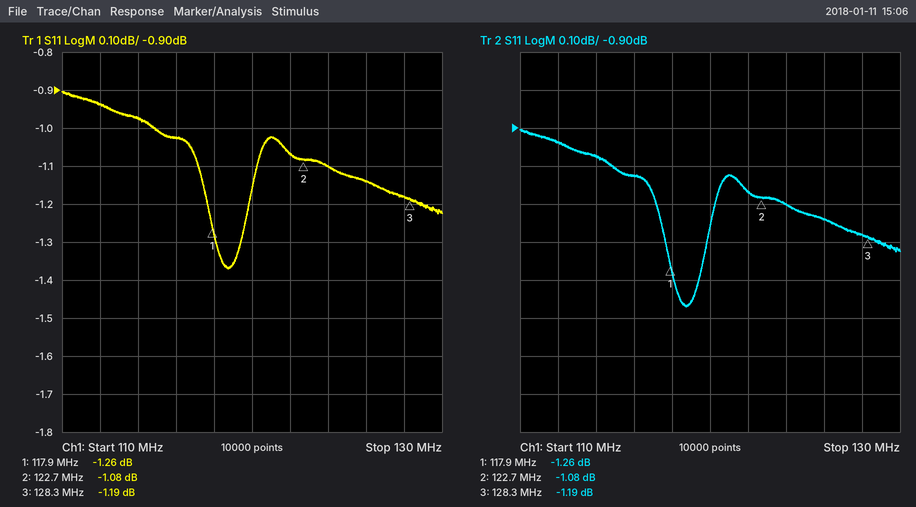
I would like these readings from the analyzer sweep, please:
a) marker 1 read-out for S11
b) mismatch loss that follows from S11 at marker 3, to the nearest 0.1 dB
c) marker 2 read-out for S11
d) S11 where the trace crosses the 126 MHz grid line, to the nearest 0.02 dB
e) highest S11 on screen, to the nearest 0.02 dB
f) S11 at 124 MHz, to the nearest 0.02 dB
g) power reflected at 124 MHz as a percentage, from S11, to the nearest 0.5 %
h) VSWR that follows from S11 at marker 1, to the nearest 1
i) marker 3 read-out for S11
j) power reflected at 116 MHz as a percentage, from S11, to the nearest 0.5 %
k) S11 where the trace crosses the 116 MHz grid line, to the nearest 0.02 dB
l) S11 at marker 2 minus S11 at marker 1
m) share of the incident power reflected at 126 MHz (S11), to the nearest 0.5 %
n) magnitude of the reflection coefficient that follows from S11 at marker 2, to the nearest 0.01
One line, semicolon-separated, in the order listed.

-1.26 dB; 6.2 dB; -1.08 dB; -1.14 dB; -0.90 dB; -1.10 dB; 77.5 %; 14; -1.19 dB; 79.0 %; -1.02 dB; 0.18 dB; 77.0 %; 0.88
